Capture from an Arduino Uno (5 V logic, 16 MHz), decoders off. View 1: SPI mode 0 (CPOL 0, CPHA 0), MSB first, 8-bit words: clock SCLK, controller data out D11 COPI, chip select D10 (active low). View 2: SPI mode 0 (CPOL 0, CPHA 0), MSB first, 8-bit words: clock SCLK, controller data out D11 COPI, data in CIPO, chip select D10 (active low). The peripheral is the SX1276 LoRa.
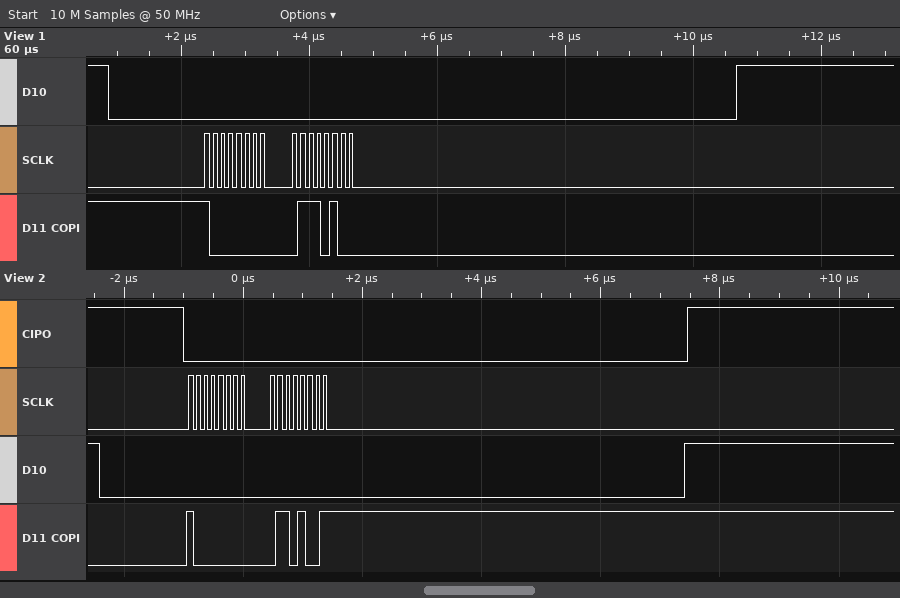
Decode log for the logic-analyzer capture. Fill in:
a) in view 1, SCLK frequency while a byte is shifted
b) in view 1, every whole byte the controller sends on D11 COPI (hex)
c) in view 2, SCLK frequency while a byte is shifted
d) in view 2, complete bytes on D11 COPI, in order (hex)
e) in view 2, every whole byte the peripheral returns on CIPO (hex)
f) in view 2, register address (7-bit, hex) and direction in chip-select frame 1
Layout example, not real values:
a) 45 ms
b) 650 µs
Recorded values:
a) 8 MHz
b) 80 74
c) 8 MHz
d) 0x80 0x69
e) 0x00 0x00
f) 0x00 write
